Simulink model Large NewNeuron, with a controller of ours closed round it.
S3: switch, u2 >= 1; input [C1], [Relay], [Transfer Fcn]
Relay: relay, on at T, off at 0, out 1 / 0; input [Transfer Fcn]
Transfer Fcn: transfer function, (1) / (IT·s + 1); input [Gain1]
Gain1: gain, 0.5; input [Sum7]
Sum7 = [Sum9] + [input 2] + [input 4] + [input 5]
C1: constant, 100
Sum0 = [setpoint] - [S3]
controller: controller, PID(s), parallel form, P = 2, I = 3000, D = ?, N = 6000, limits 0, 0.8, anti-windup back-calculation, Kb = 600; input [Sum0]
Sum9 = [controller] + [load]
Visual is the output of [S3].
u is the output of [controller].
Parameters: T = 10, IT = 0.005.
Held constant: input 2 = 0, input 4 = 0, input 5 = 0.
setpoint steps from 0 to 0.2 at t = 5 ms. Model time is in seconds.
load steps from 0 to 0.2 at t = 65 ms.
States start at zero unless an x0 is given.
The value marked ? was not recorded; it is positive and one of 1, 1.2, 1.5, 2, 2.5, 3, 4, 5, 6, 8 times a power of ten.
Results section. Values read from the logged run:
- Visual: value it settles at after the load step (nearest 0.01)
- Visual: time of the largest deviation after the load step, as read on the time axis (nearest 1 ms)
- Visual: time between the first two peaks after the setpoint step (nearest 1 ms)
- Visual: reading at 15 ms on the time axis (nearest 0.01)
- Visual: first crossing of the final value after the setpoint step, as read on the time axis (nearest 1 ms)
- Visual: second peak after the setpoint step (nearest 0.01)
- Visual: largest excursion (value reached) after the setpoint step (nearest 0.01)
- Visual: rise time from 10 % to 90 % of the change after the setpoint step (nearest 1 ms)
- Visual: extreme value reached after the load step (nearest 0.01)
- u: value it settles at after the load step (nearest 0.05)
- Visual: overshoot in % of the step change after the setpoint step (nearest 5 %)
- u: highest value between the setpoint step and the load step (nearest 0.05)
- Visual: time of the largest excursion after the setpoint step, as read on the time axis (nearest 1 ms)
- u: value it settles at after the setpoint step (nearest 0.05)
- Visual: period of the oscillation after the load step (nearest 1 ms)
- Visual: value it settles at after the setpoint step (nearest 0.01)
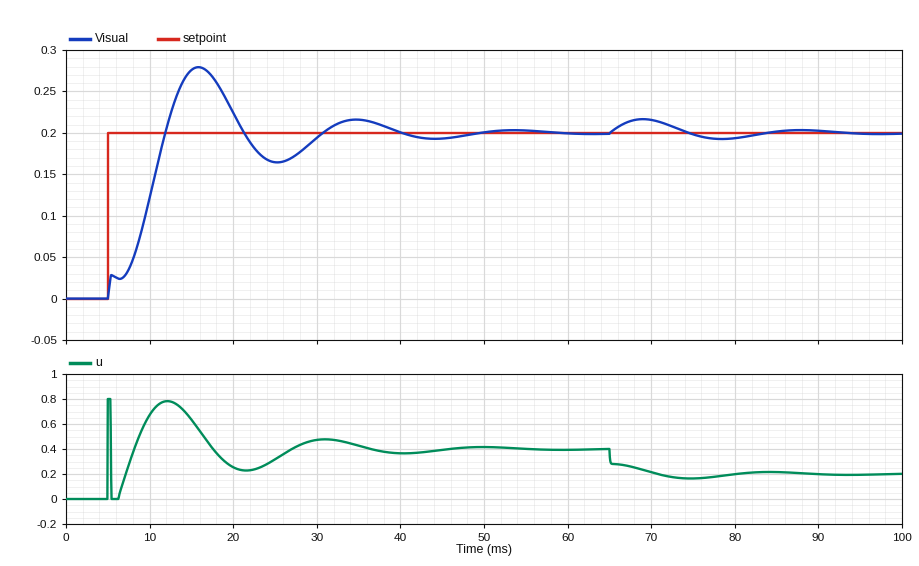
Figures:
0.20
69 ms
19 ms
0.28
12 ms
0.22
0.28
6 ms
0.22
0.20
40 %
0.80
16 ms
0.40
19 ms
0.20
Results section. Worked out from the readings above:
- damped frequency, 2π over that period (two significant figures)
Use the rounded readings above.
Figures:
0.33 rad/ms
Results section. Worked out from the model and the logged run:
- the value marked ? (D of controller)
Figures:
0.015
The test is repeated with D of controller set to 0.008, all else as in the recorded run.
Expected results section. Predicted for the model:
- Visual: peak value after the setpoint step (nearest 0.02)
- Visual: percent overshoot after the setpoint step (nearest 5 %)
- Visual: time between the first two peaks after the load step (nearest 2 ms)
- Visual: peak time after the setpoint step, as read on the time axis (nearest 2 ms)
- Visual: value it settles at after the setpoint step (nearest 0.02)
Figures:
0.26
35 %
16 ms
14 ms
0.20
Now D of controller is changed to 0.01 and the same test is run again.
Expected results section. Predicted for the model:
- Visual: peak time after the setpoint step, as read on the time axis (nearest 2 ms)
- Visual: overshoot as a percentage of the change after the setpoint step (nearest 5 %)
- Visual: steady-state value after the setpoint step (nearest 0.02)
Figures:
14 ms
35 %
0.20
